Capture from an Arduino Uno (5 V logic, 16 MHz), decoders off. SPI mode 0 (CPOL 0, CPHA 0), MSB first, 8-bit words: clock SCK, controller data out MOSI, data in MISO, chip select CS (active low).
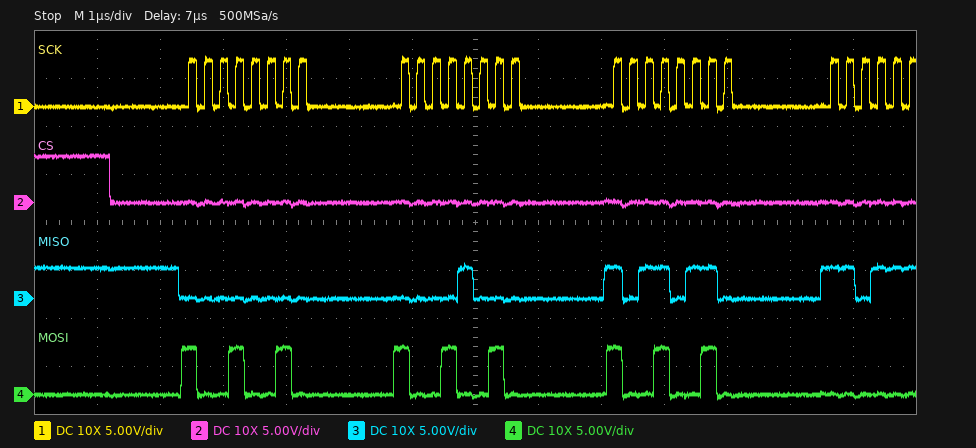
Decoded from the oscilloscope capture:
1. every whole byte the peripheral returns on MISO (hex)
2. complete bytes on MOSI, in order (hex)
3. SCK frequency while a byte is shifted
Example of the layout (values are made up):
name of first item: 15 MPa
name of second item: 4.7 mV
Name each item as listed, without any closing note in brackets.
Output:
every whole byte the peripheral returns on MISO: 00 08 B6
complete bytes on MOSI, in order: 92 92 92
SCK frequency while a byte is shifted: 4 MHz
